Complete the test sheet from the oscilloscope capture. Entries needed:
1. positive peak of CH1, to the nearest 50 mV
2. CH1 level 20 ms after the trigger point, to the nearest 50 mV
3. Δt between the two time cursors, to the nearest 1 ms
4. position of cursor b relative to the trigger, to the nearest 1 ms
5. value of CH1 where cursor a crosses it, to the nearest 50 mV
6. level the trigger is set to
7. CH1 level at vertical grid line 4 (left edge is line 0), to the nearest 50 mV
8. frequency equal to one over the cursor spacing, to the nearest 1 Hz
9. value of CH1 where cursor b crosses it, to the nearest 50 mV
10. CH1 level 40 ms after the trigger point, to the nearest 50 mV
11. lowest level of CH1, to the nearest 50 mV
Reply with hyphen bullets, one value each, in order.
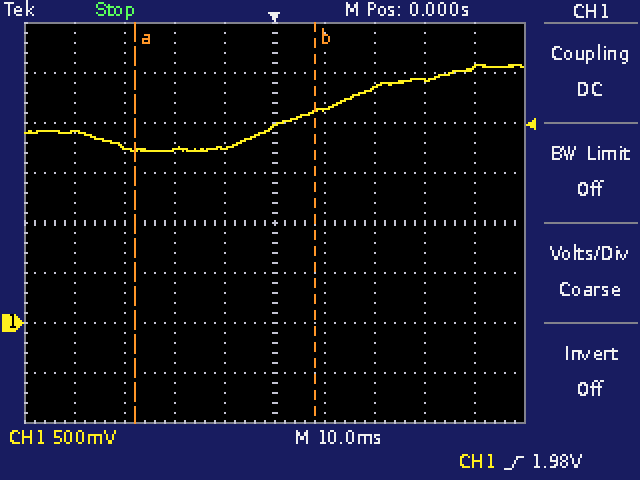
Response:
- 2.60 V
- 2.35 V
- 36 ms
- +8 ms
- 1.75 V
- 1.98 V
- 1.75 V
- 28 Hz
- 2.10 V
- 2.55 V
- 1.70 V
